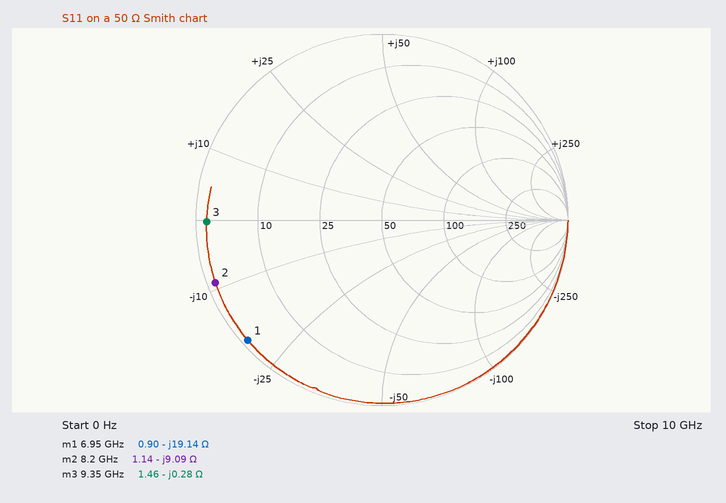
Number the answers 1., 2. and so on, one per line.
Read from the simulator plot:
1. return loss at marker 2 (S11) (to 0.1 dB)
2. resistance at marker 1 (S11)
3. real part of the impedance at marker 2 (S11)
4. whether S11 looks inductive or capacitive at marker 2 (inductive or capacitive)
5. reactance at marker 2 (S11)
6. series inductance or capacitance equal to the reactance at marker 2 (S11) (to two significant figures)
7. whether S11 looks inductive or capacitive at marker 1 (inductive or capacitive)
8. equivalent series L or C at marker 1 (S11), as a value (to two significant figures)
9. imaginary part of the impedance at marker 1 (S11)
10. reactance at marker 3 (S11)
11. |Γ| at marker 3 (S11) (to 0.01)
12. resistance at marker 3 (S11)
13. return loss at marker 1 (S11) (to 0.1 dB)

1. 0.4 dB
2. 0.90 Ω
3. 1.14 Ω
4. capacitive
5. -9.09 Ω
6. 2.1 pF
7. capacitive
8. 1.2 pF
9. -19.14 Ω
10. -0.28 Ω
11. 0.94
12. 1.46 Ω
13. 0.3 dB
